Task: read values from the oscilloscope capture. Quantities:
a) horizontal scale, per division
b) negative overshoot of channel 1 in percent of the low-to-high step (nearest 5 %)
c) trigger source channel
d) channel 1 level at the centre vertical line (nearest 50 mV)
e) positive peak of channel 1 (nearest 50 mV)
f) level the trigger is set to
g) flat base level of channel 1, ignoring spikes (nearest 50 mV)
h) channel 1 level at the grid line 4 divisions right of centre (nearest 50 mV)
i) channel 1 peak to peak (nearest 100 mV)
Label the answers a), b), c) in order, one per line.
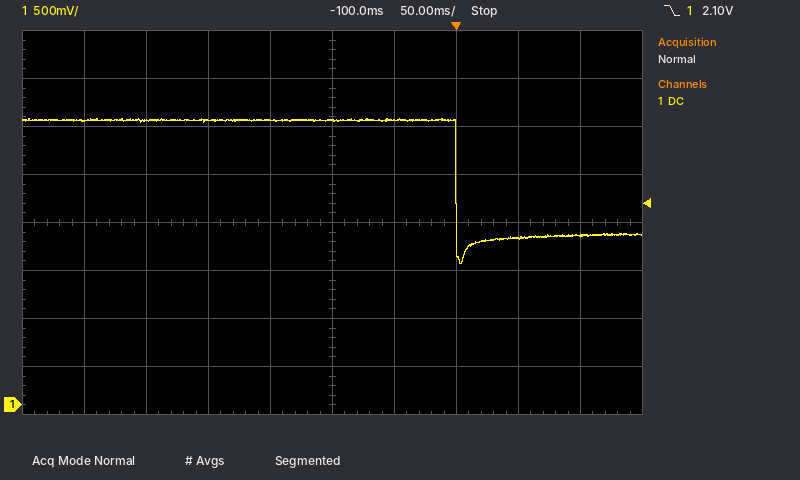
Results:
a) 50 ms
b) 25 %
c) channel 1
d) 2.95 V
e) 3.00 V
f) 2.10 V
g) 1.75 V
h) 1.75 V
i) 1.50 V
